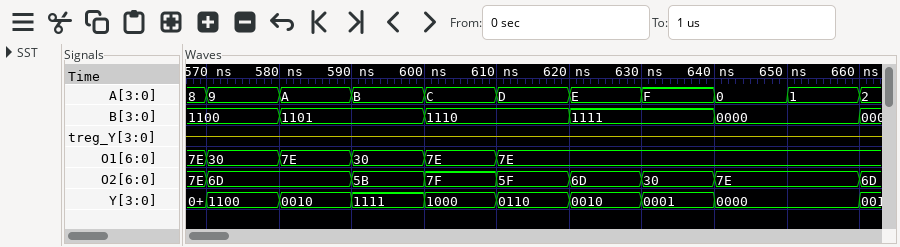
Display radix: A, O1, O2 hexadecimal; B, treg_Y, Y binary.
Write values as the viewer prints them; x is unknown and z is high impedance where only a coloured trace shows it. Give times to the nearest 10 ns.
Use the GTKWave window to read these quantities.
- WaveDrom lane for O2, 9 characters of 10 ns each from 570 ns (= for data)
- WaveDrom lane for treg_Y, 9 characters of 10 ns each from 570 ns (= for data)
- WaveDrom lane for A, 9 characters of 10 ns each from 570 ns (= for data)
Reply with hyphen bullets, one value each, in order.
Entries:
- {name: 'O2', wave: '=.======.', data: '6D 5B 7F 5F 6D 30 7E'}
- {name: 'treg_Y', wave: 'z........'}
- {name: 'A', wave: '=========', data: '9 A B C D E F 0 1'}
